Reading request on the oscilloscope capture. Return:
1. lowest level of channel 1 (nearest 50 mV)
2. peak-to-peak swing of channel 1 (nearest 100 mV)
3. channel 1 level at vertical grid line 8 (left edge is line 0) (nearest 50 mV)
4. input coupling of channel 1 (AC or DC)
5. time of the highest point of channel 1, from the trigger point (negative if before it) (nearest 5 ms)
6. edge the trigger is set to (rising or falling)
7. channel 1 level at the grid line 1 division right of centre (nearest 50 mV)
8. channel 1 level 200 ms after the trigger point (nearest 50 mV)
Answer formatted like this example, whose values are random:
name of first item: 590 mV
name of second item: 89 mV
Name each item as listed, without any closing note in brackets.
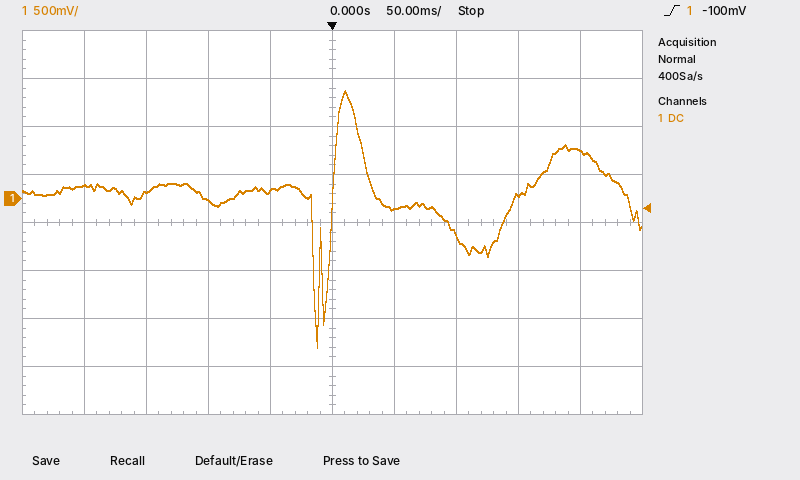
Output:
lowest level of channel 1: -1.55 V
peak-to-peak swing of channel 1: 2.70 V
channel 1 level at vertical grid line 8 (left edge is line 0): 50 mV
input coupling of channel 1: DC
time of the highest point of channel 1, from the trigger point (negative if before it): +10 ms
edge the trigger is set to: rising
channel 1 level at the grid line 1 division right of centre: -100 mV
channel 1 level 200 ms after the trigger point: 500 mV
